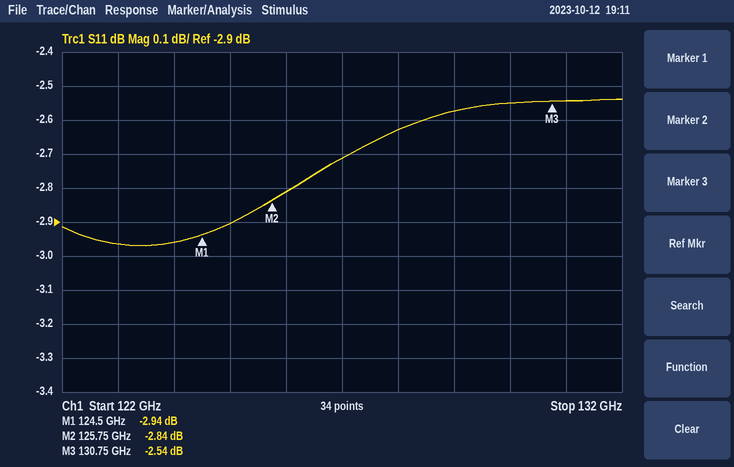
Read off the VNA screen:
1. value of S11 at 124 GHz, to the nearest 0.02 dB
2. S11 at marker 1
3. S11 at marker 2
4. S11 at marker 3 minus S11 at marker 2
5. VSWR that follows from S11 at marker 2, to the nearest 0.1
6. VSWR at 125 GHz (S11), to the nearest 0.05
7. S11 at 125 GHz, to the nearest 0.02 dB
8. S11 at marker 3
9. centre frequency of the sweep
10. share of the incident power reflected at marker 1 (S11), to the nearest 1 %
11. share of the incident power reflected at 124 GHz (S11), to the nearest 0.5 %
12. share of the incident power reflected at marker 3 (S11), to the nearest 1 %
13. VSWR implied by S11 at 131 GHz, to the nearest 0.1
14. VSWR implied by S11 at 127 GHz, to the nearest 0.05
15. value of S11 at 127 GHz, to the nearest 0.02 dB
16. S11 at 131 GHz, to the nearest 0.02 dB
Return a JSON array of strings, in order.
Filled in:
["-2.96 dB", "-2.94 dB", "-2.84 dB", "0.30 dB", "6.2", "6.05", "-2.90 dB", "-2.54 dB", "127 GHz", "51 %", "50.5 %", "56 %", "6.9", "6.45", "-2.72 dB", "-2.54 dB"]
